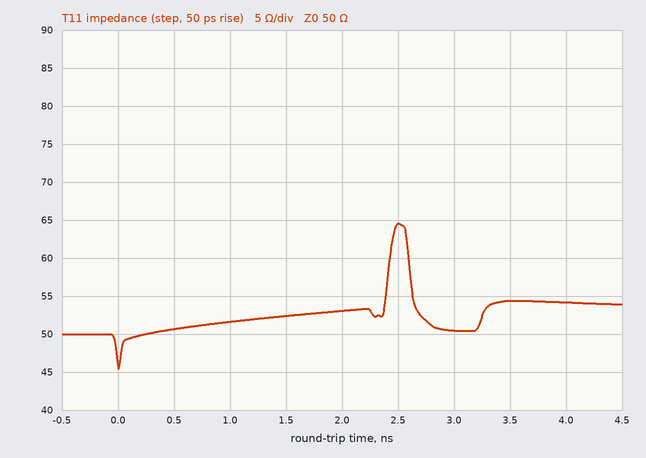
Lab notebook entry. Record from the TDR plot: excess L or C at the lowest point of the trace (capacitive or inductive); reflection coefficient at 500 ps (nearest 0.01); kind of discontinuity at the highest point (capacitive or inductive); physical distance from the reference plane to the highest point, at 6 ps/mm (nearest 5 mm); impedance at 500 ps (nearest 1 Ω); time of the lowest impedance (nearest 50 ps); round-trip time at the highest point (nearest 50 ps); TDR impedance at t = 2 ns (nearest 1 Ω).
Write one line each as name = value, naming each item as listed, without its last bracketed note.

excess L or C at the lowest point of the trace = capacitive
reflection coefficient at 500 ps = +0.01
kind of discontinuity at the highest point = inductive
physical distance from the reference plane to the highest point, at 6 ps/mm = 210 mm
impedance at 500 ps = 51 Ω
time of the lowest impedance = 0 ps
round-trip time at the highest point = 2.50 ns
TDR impedance at t = 2 ns = 53 Ω
